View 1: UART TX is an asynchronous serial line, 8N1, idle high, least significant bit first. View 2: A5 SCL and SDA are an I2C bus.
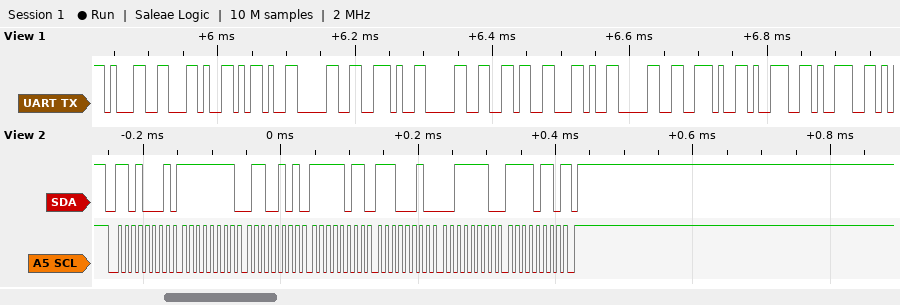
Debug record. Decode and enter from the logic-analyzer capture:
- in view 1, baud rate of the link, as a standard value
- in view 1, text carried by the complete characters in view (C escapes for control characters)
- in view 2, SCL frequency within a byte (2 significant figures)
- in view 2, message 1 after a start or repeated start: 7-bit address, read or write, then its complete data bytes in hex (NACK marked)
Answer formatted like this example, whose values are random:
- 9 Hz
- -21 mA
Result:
- 115200 baud
- "1,-0.06,0.99"
- 100 kHz
- 0x68 read: FF 65 FB E2 3E F6 NACK
